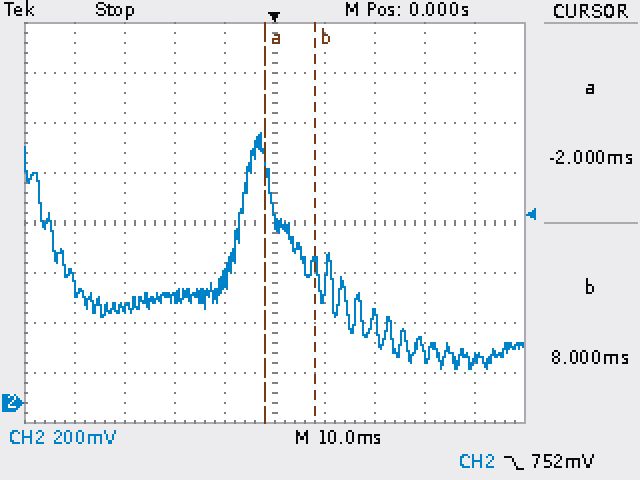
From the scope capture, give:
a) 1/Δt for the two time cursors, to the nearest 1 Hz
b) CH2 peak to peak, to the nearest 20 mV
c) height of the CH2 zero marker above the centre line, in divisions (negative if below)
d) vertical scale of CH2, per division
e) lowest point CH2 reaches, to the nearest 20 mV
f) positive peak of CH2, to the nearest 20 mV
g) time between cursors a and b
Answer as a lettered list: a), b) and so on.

a) 100 Hz
b) 940 mV
c) -3.6 div
d) 200 mV
e) 140 mV
f) 1.08 V
g) 10 ms
